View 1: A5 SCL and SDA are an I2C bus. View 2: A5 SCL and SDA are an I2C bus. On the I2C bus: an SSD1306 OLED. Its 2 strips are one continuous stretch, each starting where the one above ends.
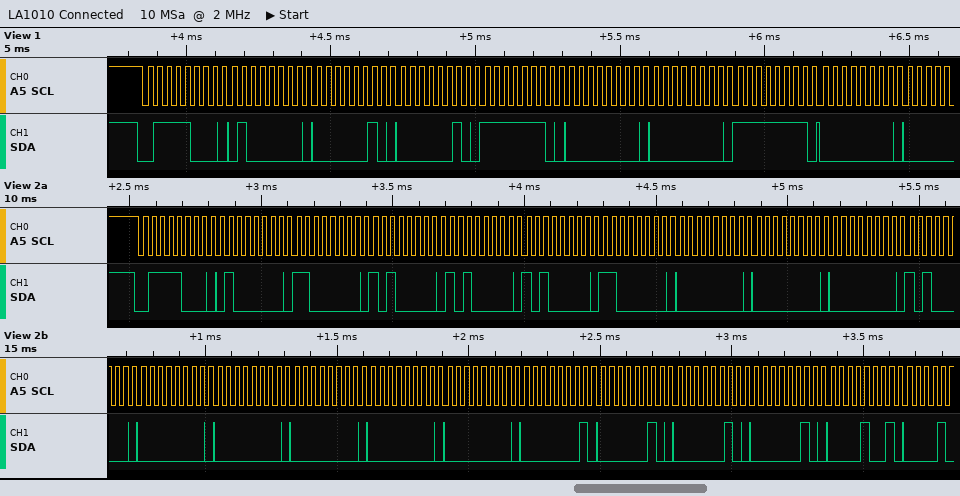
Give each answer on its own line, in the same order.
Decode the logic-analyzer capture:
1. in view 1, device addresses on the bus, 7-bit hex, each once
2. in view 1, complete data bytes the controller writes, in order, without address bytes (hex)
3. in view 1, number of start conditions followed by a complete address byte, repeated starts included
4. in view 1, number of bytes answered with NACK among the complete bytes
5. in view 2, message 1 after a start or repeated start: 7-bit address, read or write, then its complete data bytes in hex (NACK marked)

0x3C
40 02 02 FE 00 00 FF 00
1
0
0x3C write: 40 C0 A0 A0 A0 C0 00 00 00 A0 00 00 00 00 00 01 02 02 02 09
